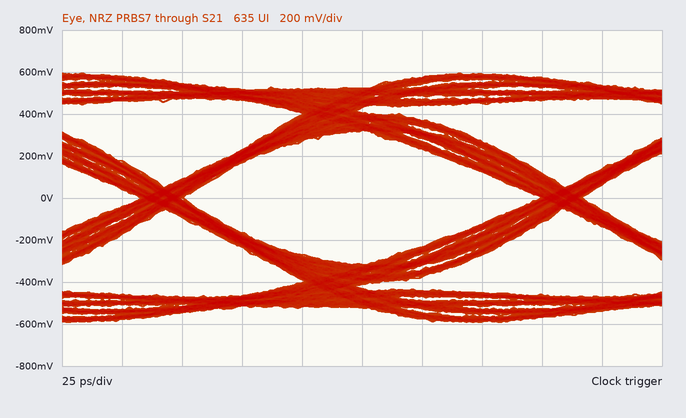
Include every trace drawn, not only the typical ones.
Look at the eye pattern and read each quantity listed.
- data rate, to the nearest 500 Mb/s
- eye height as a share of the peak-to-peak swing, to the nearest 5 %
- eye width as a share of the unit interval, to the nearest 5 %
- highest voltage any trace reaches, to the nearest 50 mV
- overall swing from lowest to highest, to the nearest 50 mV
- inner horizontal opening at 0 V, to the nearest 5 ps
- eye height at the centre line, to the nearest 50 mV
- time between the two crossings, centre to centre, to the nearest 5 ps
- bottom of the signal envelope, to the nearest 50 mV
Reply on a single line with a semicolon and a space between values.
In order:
6.0 Gb/s; 55 %; 90 %; 600 mV; 1.20 V; 150 ps; 650 mV; 165 ps; -600 mV
